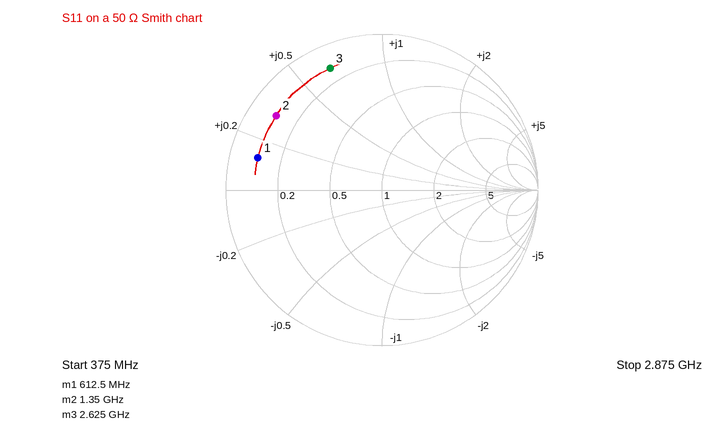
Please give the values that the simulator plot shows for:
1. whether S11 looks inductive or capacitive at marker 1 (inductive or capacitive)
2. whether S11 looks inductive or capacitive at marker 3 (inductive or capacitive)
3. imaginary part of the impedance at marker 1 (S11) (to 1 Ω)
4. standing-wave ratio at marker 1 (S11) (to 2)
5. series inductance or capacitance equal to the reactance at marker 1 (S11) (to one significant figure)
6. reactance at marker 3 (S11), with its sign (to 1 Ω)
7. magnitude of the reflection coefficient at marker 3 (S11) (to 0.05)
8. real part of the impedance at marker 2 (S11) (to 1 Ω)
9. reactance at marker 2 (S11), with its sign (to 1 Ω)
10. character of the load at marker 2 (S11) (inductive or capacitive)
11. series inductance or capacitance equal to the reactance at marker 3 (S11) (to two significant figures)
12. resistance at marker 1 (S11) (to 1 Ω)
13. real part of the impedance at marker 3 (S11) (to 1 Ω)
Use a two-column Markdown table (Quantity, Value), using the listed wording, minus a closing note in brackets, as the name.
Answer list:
| Quantity | Value |
|---|---|
| whether S11 looks inductive or capacitive at marker 1 | inductive |
| whether S11 looks inductive or capacitive at marker 3 | inductive |
| imaginary part of the impedance at marker 1 (S11) | +6 Ω |
| standing-wave ratio at marker 1 (S11) | 10 |
| series inductance or capacitance equal to the reactance at marker 1 (S11) | 2 nH |
| reactance at marker 3 (S11), with its sign | +33 Ω |
| magnitude of the reflection coefficient at marker 3 (S11) | 0.85 |
| real part of the impedance at marker 2 (S11) | 5 Ω |
| reactance at marker 2 (S11), with its sign | +16 Ω |
| character of the load at marker 2 (S11) | inductive |
| series inductance or capacitance equal to the reactance at marker 3 (S11) | 2.0 nH |
| resistance at marker 1 (S11) | 5 Ω |
| real part of the impedance at marker 3 (S11) | 6 Ω |
